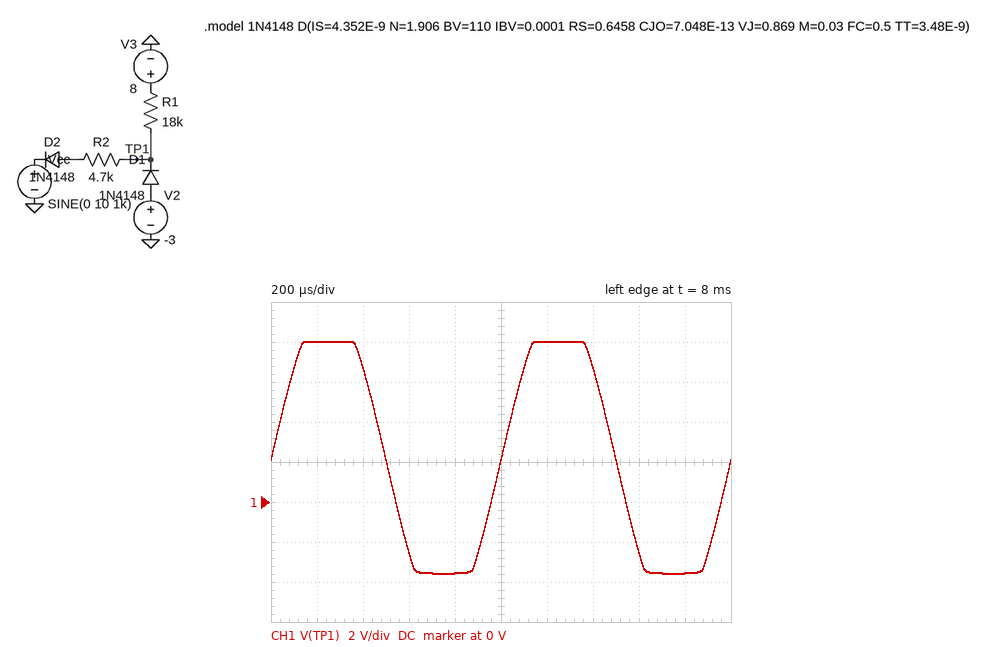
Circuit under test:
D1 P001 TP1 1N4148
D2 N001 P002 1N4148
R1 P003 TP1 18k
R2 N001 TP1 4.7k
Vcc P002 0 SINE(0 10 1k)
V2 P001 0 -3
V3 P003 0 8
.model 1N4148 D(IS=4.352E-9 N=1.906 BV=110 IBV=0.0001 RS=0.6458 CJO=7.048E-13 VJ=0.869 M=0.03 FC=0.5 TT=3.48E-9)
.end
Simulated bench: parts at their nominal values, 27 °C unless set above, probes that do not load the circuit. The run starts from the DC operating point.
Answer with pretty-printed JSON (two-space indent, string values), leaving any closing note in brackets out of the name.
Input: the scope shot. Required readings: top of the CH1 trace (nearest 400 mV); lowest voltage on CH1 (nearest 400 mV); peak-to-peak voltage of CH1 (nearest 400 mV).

{
  "top of the CH1 trace": "8.0 V",
  "lowest voltage on CH1": "-3.6 V",
  "peak-to-peak voltage of CH1": "11.6 V"
}
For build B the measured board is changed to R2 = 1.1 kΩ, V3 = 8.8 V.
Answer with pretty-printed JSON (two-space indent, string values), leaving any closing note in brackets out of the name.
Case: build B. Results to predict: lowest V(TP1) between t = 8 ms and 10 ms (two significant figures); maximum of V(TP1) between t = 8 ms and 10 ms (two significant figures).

{
  "lowest V(TP1) between t = 8 ms and 10 ms": "-3.7 V",
  "maximum of V(TP1) between t = 8 ms and 10 ms": "8.8 V"
}
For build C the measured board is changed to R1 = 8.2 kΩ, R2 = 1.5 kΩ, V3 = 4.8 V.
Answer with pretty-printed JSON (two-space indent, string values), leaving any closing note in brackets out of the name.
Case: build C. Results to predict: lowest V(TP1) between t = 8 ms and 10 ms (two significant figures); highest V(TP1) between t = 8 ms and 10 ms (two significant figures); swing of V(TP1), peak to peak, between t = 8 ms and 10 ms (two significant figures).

{
  "lowest V(TP1) between t = 8 ms and 10 ms": "-3.7 V",
  "highest V(TP1) between t = 8 ms and 10 ms": "4.8 V",
  "swing of V(TP1), peak to peak, between t = 8 ms and 10 ms": "8.5 V"
}
